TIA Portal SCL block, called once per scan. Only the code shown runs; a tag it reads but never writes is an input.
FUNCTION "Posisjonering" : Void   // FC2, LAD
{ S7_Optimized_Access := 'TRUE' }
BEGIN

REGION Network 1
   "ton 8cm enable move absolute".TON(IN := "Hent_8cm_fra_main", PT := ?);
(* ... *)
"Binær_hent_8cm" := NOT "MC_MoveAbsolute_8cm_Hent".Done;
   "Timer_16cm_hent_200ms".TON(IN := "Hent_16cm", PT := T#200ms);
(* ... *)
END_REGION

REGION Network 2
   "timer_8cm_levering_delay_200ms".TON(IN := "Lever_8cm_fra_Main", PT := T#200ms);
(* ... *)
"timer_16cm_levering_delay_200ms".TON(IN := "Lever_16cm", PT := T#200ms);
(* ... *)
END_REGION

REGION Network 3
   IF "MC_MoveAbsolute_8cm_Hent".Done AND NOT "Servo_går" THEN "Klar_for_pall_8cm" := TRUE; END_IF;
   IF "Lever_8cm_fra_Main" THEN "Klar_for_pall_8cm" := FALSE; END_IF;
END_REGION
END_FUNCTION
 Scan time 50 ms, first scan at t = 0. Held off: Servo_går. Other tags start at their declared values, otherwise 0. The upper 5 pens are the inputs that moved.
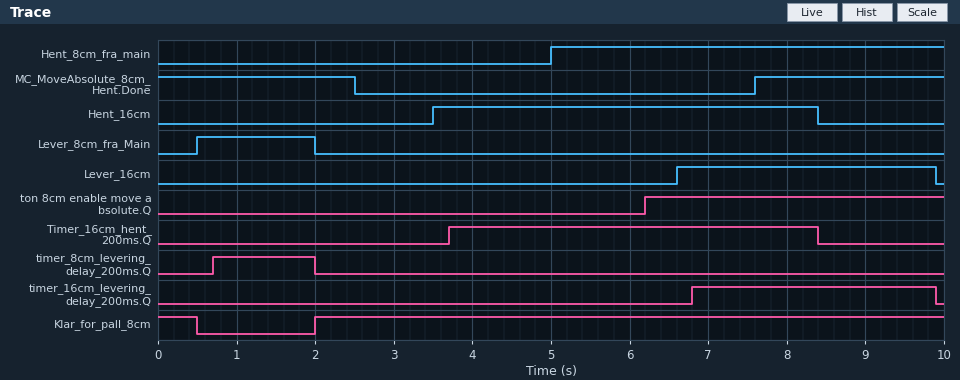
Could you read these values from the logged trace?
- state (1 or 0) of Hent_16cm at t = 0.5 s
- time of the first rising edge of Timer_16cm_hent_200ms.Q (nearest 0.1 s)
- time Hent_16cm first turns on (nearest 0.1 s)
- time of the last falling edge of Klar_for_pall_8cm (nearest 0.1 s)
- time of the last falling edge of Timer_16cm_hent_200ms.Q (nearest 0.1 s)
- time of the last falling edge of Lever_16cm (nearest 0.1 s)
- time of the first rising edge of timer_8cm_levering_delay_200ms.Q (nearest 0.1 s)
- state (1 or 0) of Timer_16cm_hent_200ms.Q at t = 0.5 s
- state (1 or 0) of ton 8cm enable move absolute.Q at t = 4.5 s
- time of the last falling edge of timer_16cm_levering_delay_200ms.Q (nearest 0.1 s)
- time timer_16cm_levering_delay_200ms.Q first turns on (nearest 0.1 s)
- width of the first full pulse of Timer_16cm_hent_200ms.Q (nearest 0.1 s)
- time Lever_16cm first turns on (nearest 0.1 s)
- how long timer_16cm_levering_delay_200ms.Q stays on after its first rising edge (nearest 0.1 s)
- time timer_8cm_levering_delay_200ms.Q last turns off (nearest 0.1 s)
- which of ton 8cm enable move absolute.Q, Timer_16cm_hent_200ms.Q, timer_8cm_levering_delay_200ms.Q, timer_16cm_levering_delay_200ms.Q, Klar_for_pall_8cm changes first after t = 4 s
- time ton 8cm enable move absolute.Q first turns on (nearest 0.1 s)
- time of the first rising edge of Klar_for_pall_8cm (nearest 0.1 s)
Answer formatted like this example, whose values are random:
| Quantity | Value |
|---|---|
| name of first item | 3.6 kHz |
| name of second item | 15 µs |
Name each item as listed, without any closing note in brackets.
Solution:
| Quantity | Value |
|---|---|
| state (1 or 0) of Hent_16cm at t = 0.5 s | 0 |
| time of the first rising edge of Timer_16cm_hent_200ms.Q | 3.7 s |
| time Hent_16cm first turns on | 3.5 s |
| time of the last falling edge of Klar_for_pall_8cm | 0.5 s |
| time of the last falling edge of Timer_16cm_hent_200ms.Q | 8.4 s |
| time of the last falling edge of Lever_16cm | 9.9 s |
| time of the first rising edge of timer_8cm_levering_delay_200ms.Q | 0.7 s |
| state (1 or 0) of Timer_16cm_hent_200ms.Q at t = 0.5 s | 0 |
| state (1 or 0) of ton 8cm enable move absolute.Q at t = 4.5 s | 0 |
| time of the last falling edge of timer_16cm_levering_delay_200ms.Q | 9.9 s |
| time timer_16cm_levering_delay_200ms.Q first turns on | 6.8 s |
| width of the first full pulse of Timer_16cm_hent_200ms.Q | 4.7 s |
| time Lever_16cm first turns on | 6.6 s |
| how long timer_16cm_levering_delay_200ms.Q stays on after its first rising edge | 3.1 s |
| time timer_8cm_levering_delay_200ms.Q last turns off | 2.0 s |
| which of ton 8cm enable move absolute.Q, Timer_16cm_hent_200ms.Q, timer_8cm_levering_delay_200ms.Q, timer_16cm_levering_delay_200ms.Q, Klar_for_pall_8cm changes first after t = 4 s | ton 8cm enable move absolute.Q |
| time ton 8cm enable move absolute.Q first turns on | 6.2 s |
| time of the first rising edge of Klar_for_pall_8cm | 2.0 s |
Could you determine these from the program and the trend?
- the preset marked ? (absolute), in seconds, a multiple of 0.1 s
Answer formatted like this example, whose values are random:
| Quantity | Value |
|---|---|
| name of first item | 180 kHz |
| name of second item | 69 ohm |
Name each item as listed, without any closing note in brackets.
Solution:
| Quantity | Value |
|---|---|
| the preset marked ? (absolute), in seconds, a multiple of 0.1 s | 1.2 s |
